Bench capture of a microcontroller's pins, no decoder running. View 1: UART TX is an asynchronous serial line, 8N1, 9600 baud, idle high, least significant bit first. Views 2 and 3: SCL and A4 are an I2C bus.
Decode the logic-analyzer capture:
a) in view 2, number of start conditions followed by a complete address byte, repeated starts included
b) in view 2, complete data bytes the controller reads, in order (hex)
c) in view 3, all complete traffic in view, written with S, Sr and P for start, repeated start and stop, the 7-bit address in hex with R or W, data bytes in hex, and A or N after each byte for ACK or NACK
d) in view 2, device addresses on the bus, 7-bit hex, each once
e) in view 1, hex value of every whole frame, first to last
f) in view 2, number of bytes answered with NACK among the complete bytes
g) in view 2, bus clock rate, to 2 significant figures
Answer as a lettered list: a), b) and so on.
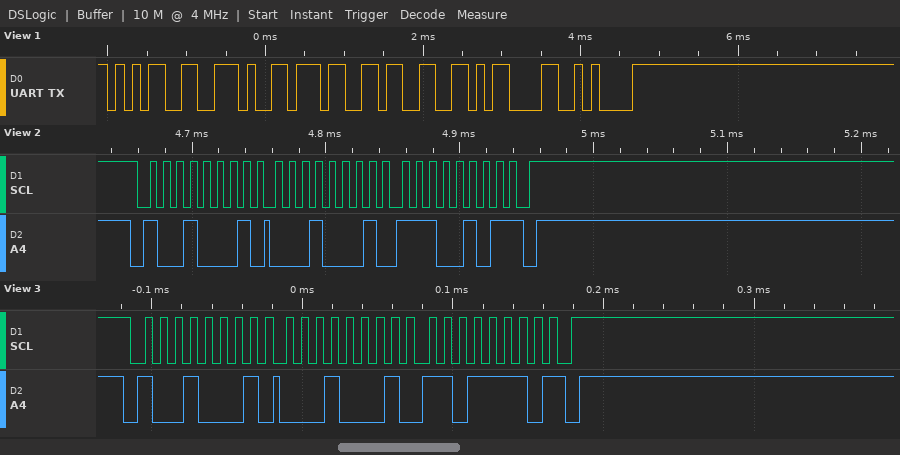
a) 1
b) 11 E5
c) S 48R A 11 A DE N P
d) 0x48
e) 0x35 0x2E 0x37 0x33 0x0D 0x0A
f) 1
g) 100 kHz
